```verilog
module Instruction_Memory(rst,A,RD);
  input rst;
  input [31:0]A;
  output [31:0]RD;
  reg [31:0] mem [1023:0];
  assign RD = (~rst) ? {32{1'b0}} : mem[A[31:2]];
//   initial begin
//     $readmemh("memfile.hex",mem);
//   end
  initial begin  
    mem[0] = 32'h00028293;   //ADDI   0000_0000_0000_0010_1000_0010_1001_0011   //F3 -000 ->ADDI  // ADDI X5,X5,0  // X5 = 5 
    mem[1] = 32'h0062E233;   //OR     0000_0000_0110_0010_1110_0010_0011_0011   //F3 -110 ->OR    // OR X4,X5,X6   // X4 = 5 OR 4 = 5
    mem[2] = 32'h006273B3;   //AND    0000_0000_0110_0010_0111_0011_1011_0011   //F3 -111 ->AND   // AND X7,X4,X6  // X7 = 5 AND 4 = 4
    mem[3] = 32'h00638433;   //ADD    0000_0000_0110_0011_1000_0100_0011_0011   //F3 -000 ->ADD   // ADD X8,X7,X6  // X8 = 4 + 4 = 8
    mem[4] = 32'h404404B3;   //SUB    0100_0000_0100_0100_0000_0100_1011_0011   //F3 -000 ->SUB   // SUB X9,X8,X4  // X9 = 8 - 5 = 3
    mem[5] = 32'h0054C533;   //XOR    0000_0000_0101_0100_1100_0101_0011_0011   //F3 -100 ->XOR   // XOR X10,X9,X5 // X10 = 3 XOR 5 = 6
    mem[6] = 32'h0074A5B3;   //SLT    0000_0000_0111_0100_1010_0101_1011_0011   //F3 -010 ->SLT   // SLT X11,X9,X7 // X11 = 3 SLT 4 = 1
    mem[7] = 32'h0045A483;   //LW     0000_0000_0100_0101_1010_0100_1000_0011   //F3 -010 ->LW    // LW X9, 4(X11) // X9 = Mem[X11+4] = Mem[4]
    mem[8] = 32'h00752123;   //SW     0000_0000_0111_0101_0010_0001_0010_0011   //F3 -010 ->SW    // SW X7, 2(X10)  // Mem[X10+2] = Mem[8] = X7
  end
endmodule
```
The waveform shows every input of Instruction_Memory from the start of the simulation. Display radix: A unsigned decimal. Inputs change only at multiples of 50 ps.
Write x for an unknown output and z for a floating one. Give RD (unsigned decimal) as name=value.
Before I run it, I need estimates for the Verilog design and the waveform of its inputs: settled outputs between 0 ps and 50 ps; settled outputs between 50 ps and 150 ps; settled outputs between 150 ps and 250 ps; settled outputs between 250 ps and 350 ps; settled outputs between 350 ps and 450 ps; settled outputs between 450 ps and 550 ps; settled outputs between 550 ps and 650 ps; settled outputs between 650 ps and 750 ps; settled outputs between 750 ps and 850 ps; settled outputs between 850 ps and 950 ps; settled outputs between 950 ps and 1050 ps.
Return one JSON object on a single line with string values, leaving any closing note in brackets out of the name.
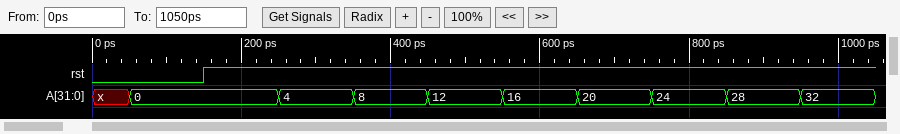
{"settled outputs between 0 ps and 50 ps": "RD=0", "settled outputs between 50 ps and 150 ps": "RD=0", "settled outputs between 150 ps and 250 ps": "RD=164499", "settled outputs between 250 ps and 350 ps": "RD=6480435", "settled outputs between 350 ps and 450 ps": "RD=6452147", "settled outputs between 450 ps and 550 ps": "RD=6521907", "settled outputs between 550 ps and 650 ps": "RD=1078199475", "settled outputs between 650 ps and 750 ps": "RD=5555507", "settled outputs between 750 ps and 850 ps": "RD=7644595", "settled outputs between 850 ps and 950 ps": "RD=4564099", "settled outputs between 950 ps and 1050 ps": "RD=7676195"}
